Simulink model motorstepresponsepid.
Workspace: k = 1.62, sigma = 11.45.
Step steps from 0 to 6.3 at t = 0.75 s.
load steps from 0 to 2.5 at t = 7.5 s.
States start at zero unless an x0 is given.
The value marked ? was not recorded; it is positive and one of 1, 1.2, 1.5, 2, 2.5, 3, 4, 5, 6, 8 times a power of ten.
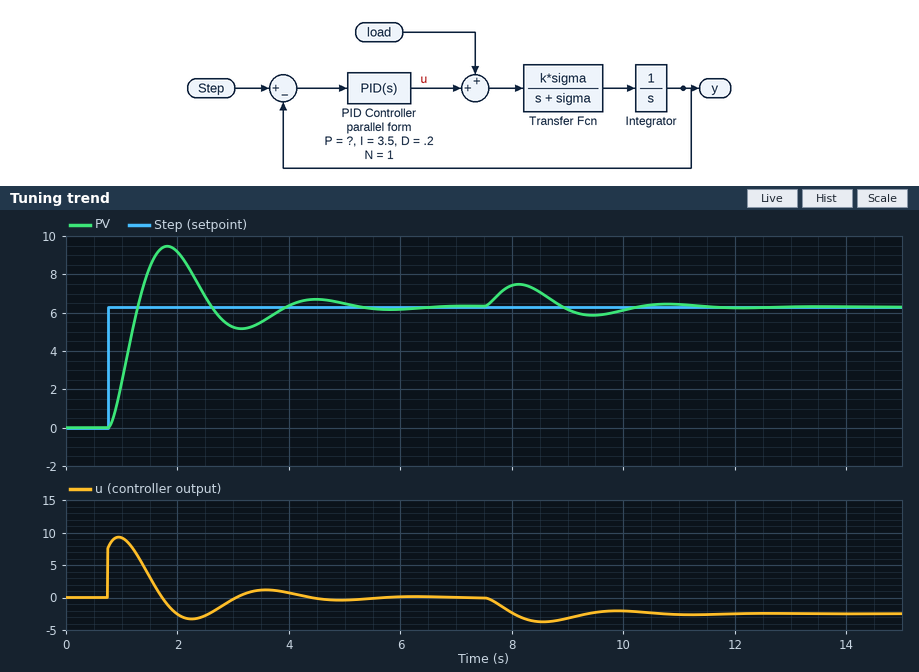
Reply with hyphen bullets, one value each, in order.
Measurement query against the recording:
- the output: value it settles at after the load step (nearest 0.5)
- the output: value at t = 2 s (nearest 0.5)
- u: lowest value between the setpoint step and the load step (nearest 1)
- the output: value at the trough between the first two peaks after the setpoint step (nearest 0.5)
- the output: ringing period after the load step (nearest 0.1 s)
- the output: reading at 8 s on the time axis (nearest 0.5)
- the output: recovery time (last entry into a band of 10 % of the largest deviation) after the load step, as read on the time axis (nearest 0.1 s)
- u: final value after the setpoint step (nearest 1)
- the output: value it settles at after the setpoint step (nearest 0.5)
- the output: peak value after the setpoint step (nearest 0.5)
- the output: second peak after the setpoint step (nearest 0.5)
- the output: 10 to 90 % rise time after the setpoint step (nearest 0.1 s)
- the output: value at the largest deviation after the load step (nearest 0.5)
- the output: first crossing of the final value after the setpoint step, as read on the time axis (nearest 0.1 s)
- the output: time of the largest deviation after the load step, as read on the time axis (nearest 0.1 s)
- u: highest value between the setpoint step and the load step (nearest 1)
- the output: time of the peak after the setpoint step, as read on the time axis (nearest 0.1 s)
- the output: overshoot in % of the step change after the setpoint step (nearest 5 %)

- 6.5
- 9.0
- -3
- 5.0
- 2.7 s
- 7.5
- 11.1 s
- 0
- 6.5
- 9.5
- 6.5
- 0.4 s
- 7.5
- 1.3 s
- 8.1 s
- 9
- 1.8 s
- 50 %
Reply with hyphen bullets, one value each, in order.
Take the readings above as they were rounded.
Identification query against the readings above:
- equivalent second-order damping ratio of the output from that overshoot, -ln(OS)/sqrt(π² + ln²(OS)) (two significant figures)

- 0.22
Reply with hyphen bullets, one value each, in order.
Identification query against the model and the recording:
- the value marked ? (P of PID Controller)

- 1
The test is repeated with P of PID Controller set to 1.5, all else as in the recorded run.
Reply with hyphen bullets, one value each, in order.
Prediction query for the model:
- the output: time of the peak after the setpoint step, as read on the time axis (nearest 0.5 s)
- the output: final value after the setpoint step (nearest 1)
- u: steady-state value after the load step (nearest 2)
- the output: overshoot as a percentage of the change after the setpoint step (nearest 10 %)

- 1.5 s
- 6
- -2
- 40 %
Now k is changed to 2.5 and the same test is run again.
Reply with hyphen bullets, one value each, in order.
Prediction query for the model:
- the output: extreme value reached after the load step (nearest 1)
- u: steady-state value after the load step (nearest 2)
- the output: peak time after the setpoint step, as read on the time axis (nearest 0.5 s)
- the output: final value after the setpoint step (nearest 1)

- 8
- -2
- 1.5 s
- 6
